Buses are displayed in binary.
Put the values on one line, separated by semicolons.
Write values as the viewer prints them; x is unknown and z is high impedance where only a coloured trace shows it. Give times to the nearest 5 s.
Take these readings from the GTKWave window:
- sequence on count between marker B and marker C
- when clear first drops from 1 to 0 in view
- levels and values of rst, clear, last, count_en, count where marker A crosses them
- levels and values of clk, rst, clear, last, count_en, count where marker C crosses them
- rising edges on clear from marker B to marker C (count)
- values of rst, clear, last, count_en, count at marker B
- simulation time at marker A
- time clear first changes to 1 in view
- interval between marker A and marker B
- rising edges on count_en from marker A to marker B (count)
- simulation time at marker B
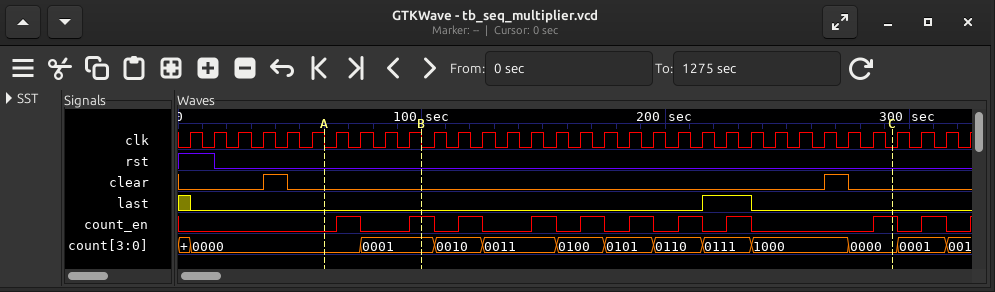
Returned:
0001, 0010, 0011, 0100, 0101, 0110, 0111, 1000, 0000; 45 s; rst=0, clear=0, last=0, count_en=0, count=0000; clk=0, rst=0, clear=0, last=0, count_en=1, count=0000; 1; rst=0, clear=0, last=0, count_en=1, count=0001; 60 s; 35 s; 40 s; 2; 100 s
